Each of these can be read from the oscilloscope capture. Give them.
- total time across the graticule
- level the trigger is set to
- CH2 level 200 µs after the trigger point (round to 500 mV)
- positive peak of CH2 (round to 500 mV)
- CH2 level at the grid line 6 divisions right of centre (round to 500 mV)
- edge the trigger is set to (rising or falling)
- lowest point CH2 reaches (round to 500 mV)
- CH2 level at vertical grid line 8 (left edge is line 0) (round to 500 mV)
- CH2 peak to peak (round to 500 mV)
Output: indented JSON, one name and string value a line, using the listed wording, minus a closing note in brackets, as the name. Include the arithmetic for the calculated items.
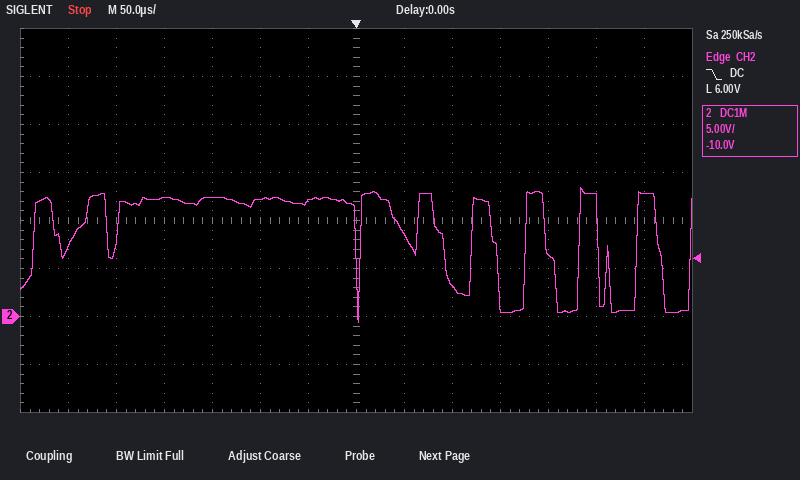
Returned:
{
  "total time across the graticule": "700 µs",
  "level the trigger is set to": "6.00 V",
  "CH2 level 200 µs after the trigger point": "6.5 V",
  "positive peak of CH2": "13.5 V",
  "CH2 level at the grid line 6 divisions right of centre": "13.0 V",
  "edge the trigger is set to": "falling",
  "lowest point CH2 reaches": "-500 mV",
  "CH2 level at vertical grid line 8 (left edge is line 0)": "8.5 V",
  "CH2 peak to peak": "13.5 V − (-500 mV) = 14.0 V"
}
